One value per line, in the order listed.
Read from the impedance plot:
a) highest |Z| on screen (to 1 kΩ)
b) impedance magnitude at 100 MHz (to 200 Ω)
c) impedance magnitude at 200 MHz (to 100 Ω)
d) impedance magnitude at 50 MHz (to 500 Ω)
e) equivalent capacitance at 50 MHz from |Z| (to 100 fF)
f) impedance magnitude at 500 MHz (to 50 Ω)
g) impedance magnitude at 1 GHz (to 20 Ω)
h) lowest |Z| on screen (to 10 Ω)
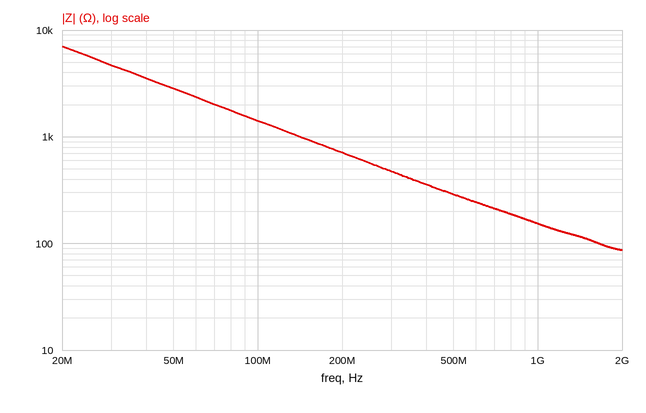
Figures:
7 kΩ
1.4 kΩ
700 Ω
3.0 kΩ
1.1 pF
300 Ω
160 Ω
90 Ω
